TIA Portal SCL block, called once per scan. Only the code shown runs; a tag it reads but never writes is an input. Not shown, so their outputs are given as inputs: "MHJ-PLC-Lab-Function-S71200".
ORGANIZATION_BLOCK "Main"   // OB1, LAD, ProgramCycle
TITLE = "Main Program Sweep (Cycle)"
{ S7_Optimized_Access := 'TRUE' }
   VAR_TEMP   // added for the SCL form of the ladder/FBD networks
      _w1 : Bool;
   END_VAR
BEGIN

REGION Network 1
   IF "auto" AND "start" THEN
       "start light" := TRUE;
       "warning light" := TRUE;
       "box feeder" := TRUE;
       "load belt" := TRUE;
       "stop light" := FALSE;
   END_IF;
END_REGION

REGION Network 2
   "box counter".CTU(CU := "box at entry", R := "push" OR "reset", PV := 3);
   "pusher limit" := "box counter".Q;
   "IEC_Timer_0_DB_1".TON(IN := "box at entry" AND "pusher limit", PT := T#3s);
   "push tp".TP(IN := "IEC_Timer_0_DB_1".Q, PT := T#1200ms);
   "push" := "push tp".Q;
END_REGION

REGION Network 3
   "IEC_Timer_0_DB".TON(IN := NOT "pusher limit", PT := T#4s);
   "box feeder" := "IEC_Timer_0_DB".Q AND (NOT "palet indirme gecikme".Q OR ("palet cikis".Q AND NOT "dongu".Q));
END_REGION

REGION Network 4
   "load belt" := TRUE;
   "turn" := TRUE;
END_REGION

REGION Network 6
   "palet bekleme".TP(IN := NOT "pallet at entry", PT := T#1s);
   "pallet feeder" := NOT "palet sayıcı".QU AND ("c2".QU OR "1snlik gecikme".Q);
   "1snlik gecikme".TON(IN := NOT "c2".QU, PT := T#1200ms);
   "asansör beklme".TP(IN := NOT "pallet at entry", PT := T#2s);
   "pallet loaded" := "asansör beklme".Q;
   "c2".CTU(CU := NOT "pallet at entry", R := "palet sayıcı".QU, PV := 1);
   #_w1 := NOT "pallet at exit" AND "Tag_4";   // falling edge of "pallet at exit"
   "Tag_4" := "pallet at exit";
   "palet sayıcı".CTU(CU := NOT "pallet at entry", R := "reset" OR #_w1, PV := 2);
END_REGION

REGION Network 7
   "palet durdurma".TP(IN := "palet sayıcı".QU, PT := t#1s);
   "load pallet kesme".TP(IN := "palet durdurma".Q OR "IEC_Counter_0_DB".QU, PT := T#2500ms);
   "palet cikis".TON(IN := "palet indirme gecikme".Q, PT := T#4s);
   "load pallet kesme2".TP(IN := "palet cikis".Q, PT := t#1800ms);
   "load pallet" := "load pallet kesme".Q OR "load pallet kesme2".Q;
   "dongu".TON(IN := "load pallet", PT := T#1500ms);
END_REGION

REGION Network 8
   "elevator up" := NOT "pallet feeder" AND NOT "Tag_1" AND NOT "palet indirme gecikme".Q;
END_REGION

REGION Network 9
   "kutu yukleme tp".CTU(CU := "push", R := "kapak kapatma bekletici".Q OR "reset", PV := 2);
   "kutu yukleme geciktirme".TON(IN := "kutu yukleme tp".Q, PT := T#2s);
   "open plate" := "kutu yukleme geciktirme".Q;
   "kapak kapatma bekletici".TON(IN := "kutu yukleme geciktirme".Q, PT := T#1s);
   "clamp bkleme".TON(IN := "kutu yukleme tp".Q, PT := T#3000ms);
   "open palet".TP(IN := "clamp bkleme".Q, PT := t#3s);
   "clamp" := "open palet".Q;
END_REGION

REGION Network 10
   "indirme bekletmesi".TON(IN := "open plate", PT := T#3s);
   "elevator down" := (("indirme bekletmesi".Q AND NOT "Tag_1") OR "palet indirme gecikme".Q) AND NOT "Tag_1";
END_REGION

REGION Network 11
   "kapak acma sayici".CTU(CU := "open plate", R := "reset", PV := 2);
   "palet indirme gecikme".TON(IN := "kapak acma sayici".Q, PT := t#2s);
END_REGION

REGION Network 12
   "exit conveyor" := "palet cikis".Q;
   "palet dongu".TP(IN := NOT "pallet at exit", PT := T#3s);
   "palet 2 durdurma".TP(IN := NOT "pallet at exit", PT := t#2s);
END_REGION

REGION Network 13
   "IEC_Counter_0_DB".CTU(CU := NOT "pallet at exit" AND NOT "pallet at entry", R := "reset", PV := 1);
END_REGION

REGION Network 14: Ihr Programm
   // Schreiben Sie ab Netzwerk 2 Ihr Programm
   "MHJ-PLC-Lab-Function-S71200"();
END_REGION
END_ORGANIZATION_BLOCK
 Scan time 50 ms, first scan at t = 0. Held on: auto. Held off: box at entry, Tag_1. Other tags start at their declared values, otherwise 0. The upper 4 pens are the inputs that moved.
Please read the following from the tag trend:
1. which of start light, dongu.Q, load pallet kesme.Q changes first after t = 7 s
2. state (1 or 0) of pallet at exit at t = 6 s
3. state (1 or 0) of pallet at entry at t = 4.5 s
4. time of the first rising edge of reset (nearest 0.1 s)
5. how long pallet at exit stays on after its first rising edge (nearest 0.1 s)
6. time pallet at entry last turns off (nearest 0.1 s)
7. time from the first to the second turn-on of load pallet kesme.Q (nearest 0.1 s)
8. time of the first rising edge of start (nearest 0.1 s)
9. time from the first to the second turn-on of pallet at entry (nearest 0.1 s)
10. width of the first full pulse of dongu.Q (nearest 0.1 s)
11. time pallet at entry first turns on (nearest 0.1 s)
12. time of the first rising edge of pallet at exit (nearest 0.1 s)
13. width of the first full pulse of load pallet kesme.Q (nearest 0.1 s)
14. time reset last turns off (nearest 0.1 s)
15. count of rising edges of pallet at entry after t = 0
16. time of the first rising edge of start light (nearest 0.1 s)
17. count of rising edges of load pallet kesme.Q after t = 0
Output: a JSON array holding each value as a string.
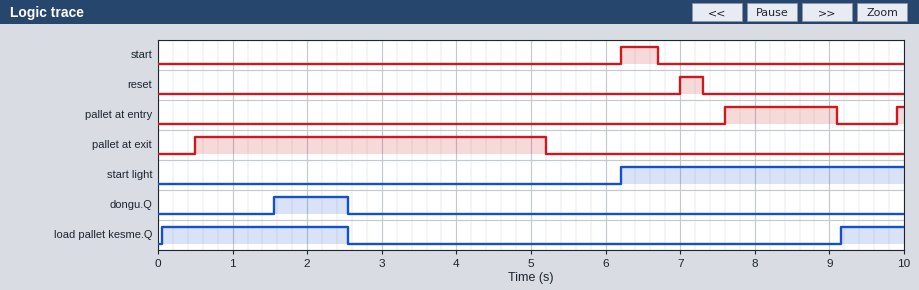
["load pallet kesme.Q", "0", "0", "7.0 s", "4.7 s", "9.1 s", "9.1 s", "6.2 s", "2.3 s", "1.0 s", "7.6 s", "0.5 s", "2.5 s", "7.3 s", "2", "6.2 s", "2"]
